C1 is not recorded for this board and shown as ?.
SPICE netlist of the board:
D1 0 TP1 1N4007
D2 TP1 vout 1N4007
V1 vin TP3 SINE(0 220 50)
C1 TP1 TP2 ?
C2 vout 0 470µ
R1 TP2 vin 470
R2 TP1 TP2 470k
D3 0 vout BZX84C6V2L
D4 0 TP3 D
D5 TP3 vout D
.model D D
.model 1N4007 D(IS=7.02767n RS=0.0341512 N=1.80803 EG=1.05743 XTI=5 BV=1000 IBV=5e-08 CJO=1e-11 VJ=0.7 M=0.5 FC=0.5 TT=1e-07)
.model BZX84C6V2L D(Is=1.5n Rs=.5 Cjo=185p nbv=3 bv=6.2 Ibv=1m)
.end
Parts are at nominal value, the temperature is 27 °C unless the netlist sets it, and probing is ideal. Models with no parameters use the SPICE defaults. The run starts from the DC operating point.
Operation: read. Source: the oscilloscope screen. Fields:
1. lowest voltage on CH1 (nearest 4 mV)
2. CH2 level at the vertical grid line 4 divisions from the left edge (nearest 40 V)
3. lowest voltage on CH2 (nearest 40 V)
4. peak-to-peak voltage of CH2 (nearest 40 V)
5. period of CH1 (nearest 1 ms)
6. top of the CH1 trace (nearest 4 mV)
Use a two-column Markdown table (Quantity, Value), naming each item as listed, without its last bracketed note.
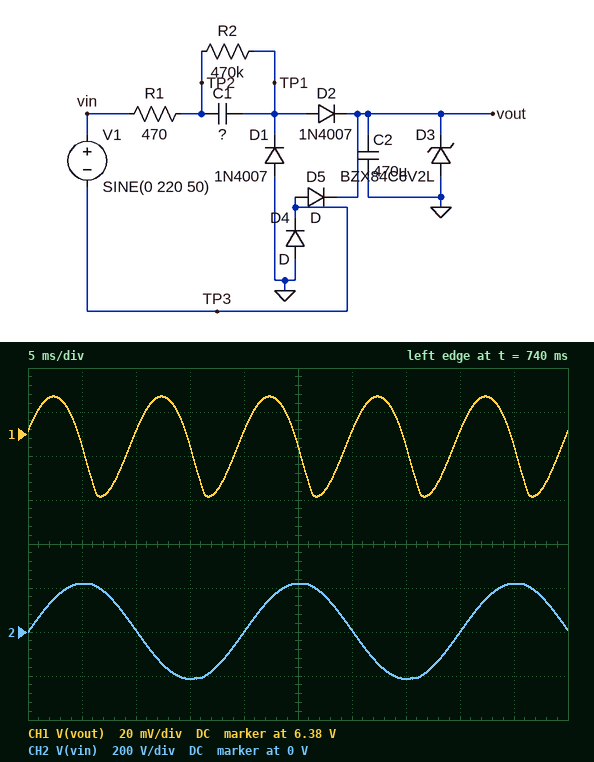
| Quantity | Value |
|---|---|
| lowest voltage on CH1 | 6.352 V |
| CH2 level at the vertical grid line 4 divisions from the left edge | 0 V |
| lowest voltage on CH2 | -200 V |
| peak-to-peak voltage of CH2 | 440 V |
| period of CH1 | 10 ms |
| top of the CH1 trace | 6.396 V |
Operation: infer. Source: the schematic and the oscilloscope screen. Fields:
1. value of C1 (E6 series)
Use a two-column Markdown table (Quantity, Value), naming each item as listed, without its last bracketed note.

| Quantity | Value |
|---|---|
| value of C1 | 220 nF |
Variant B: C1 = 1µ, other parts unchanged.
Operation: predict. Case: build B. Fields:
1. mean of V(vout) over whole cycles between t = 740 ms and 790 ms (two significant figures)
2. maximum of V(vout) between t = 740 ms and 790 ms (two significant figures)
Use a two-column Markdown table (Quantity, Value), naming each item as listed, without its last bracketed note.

| Quantity | Value |
|---|---|
| mean of V(vout) over whole cycles between t = 740 ms and 790 ms | 6.5 V |
| maximum of V(vout) between t = 740 ms and 790 ms | 6.6 V |
